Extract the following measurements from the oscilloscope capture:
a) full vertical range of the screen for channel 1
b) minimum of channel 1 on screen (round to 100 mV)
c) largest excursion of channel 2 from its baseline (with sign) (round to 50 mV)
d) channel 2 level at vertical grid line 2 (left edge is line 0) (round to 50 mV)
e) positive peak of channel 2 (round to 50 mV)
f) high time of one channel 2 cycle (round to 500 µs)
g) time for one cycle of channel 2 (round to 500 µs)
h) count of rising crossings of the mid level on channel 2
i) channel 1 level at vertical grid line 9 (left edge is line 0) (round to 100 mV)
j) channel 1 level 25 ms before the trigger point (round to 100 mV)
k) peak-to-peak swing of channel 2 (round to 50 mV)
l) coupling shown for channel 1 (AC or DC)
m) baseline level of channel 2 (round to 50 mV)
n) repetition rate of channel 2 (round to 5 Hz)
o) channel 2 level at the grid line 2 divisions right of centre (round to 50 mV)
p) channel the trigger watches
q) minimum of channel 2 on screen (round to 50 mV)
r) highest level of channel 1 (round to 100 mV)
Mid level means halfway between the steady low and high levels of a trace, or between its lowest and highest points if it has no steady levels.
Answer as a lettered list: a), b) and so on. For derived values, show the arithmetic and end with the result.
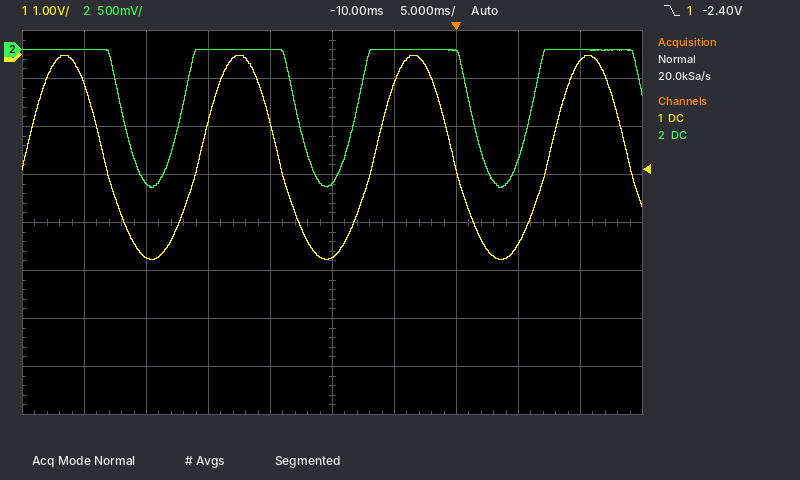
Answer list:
a) 8 V
b) -4.3 V
c) -1.45 V − (0 mV) = -1.45 V
d) -1.40 V
e) 0 mV
f) 9.5 ms
g) 14.0 ms
h) 3
i) -100 mV
j) -4.2 V
k) 0 mV − (-1.45 V) = 1.45 V
l) DC
m) 0 mV
n) 1 / 14.0 ms ≈ 71.4 Hz, so 70 Hz to the nearest 5 Hz
o) -50 mV
p) channel 1
q) -1.45 V
r) 0.0 V
